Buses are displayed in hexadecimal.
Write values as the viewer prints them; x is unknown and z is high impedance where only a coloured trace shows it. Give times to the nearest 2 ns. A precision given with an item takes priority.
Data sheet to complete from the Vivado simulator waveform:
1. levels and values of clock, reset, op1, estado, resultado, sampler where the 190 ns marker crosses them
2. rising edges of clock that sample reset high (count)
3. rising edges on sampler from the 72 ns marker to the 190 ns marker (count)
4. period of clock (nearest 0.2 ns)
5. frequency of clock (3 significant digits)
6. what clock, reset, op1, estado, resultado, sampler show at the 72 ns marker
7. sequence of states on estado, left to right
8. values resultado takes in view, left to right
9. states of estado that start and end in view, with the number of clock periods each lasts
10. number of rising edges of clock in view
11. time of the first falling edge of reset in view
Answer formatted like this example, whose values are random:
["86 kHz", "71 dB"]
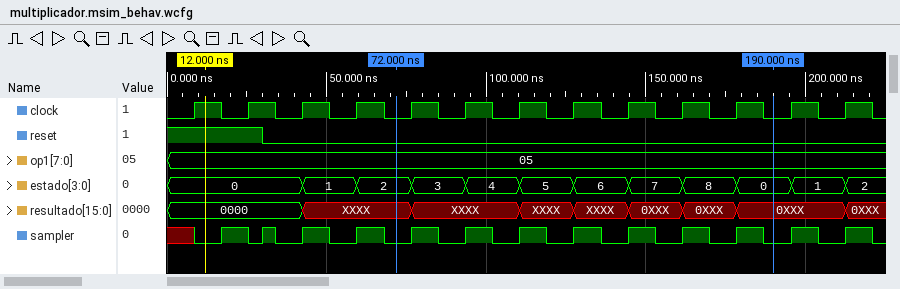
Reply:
["clock=0, reset=0, op1=05, estado=0, resultado=0XXX, sampler=0", "2", "7", "17 ns", "58.8 MHz", "clock=0, reset=0, op1=05, estado=2, resultado=XXXX, sampler=0", "0, 1, 2, 3, 4, 5, 6, 7, 8, 0, 1, 2", "0000, XXXX, XXXX, XXXX, XXXX, 0XXX, 0XXX, 0XXX, 0XXX", "1: 1, 2: 1, 3: 1, 4: 1, 5: 1, 6: 1, 7: 1, 8: 1, 0: 1, 1: 1", "13", "30 ns"]
